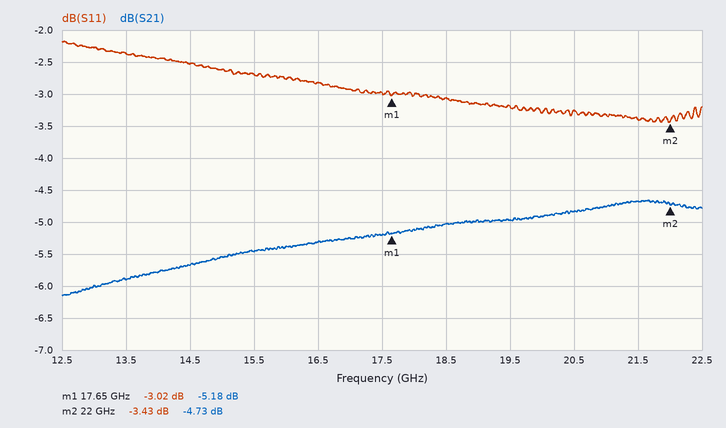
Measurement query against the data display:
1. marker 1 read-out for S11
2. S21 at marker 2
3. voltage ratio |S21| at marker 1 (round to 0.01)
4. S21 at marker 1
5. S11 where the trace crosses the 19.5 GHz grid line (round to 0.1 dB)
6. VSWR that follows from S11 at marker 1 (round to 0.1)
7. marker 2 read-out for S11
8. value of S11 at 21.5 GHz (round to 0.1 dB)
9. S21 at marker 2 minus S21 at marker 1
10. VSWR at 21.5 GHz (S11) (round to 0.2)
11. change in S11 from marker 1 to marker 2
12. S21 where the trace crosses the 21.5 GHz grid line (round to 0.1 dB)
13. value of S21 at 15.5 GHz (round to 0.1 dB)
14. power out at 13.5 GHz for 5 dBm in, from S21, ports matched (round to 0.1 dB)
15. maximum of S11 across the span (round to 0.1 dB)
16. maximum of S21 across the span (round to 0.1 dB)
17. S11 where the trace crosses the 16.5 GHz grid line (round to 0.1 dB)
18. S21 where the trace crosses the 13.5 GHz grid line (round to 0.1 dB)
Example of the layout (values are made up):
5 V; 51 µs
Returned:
-3.02 dB; -4.73 dB; 0.55; -5.18 dB; -3.2 dB; 5.8; -3.43 dB; -3.4 dB; 0.45 dB; 5.2; -0.41 dB; -4.7 dB; -5.5 dB; -0.9 dBm; -2.2 dB; -4.7 dB; -2.8 dB; -5.9 dB
